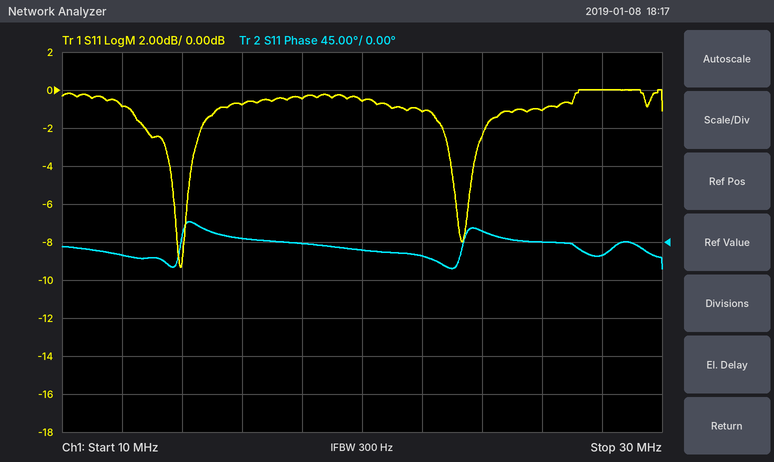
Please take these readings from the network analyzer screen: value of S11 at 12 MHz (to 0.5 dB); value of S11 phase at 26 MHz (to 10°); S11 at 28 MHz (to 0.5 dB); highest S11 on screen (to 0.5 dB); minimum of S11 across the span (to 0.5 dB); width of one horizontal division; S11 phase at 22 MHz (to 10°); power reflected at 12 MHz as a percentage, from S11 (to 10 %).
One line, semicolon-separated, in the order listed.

-1.0 dB; 0°; 0.0 dB; 0.0 dB; -9.5 dB; 2 MHz; -20°; 80 %
